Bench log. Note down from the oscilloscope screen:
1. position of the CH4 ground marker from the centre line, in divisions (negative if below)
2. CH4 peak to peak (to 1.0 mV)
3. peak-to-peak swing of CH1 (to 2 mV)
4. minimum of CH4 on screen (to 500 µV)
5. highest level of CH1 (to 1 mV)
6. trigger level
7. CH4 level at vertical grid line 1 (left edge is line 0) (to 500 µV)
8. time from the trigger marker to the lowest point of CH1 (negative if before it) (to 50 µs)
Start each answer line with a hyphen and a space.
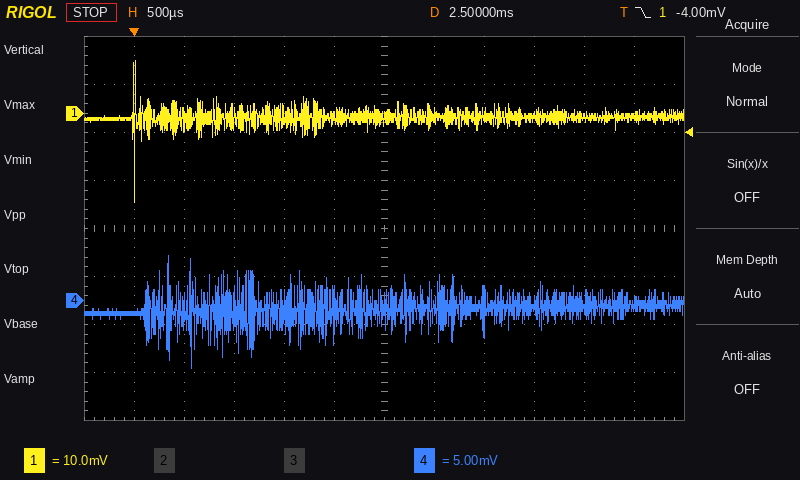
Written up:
- -1.5 div
- 12.0 mV
- 30 mV
- -7.0 mV
- 11 mV
- -4.00 mV
- -1.5 mV
- 0 µs
